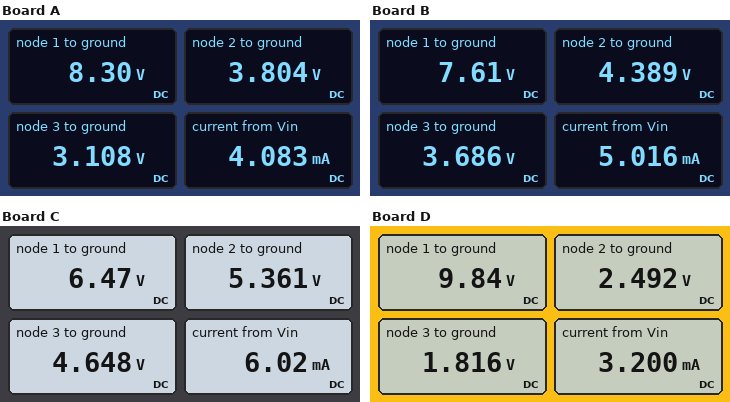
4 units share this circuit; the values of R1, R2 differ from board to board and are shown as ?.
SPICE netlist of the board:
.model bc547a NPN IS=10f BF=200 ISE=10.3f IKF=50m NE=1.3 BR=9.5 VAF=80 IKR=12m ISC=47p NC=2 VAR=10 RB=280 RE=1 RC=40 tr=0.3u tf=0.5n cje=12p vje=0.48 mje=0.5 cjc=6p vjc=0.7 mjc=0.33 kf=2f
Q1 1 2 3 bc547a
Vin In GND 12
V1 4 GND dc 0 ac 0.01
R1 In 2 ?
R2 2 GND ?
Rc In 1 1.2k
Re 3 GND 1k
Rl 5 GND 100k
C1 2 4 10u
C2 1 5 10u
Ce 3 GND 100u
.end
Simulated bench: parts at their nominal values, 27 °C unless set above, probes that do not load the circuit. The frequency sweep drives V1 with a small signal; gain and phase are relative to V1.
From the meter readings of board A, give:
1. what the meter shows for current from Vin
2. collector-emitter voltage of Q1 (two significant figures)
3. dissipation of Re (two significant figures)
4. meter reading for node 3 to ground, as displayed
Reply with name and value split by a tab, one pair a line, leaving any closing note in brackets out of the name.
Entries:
what the meter shows for current from Vin	4.083 mA
collector-emitter voltage of Q1	5.2 V
dissipation of Re	9.7 mW
meter reading for node 3 to ground, as displayed	3.108 V
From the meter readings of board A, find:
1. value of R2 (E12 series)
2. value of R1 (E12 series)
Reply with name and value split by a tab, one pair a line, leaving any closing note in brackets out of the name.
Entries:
value of R2	3.9 kΩ
value of R1	8.2 kΩ
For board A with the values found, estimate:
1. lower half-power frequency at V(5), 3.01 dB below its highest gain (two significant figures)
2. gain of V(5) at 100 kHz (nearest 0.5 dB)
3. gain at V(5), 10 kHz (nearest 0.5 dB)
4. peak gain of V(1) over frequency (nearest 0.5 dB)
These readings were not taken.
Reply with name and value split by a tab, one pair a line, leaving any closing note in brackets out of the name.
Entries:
lower half-power frequency at V(5), 3.01 dB below its highest gain	140 Hz
gain of V(5) at 100 kHz	39.5 dB
gain at V(5), 10 kHz	39.5 dB
peak gain of V(1) over frequency	39.5 dB
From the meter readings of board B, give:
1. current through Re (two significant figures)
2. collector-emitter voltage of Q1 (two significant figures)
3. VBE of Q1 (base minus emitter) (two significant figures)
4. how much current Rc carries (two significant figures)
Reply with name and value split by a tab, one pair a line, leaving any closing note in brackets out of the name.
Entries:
current through Re	3.7 mA
collector-emitter voltage of Q1	3.9 V
VBE of Q1 (base minus emitter)	700 mV
how much current Rc carries	3.7 mA
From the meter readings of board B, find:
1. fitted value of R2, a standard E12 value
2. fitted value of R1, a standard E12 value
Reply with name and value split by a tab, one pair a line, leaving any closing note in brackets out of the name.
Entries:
fitted value of R2, a standard E12 value	3.3 kΩ
fitted value of R1, a standard E12 value	5.6 kΩ
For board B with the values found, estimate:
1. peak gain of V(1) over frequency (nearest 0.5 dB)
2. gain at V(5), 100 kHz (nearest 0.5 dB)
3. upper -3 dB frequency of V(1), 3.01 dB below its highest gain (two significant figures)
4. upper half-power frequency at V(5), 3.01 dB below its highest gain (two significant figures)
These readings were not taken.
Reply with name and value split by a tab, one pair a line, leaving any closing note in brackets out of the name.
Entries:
peak gain of V(1) over frequency	40.5 dB
gain at V(5), 100 kHz	40.5 dB
upper -3 dB frequency of V(1), 3.01 dB below its highest gain	1.3 MHz
upper half-power frequency at V(5), 3.01 dB below its highest gain	1.3 MHz
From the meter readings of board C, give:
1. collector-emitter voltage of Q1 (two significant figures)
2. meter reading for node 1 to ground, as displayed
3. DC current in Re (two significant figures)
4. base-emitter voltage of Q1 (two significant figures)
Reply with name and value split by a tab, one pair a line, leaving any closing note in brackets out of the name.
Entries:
collector-emitter voltage of Q1	1.8 V
meter reading for node 1 to ground, as displayed	6.47 V
DC current in Re	4.6 mA
base-emitter voltage of Q1	710 mV
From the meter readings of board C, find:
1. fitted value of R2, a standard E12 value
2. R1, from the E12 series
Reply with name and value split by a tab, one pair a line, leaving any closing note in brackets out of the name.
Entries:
fitted value of R2, a standard E12 value	3.9 kΩ
R1, from the E12 series	4.7 kΩ
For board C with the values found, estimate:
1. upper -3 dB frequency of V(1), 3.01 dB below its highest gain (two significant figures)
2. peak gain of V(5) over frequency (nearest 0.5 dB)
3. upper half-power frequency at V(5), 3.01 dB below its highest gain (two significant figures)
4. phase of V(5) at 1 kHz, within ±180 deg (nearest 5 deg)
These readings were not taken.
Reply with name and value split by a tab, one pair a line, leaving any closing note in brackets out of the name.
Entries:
upper -3 dB frequency of V(1), 3.01 dB below its highest gain	890 kHz
peak gain of V(5) over frequency	41.5 dB
upper half-power frequency at V(5), 3.01 dB below its highest gain	890 kHz
phase of V(5) at 1 kHz, within ±180 deg	-170 deg
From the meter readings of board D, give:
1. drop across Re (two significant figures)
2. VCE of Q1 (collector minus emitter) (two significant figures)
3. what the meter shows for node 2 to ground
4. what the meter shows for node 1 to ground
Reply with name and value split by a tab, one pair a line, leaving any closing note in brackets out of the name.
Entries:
drop across Re	1.8 V
VCE of Q1 (collector minus emitter)	8.0 V
what the meter shows for node 2 to ground	2.492 V
what the meter shows for node 1 to ground	9.84 V
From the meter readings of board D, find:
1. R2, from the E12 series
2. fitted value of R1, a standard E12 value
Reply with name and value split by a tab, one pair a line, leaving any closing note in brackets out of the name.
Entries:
R2, from the E12 series	1.8 kΩ
fitted value of R1, a standard E12 value	6.8 kΩ
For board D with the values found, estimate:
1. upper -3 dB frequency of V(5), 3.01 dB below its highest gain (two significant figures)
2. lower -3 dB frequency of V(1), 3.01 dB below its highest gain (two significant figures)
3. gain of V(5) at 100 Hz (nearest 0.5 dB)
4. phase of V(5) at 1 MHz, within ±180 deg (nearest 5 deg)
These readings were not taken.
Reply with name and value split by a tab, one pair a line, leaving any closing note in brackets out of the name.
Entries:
upper -3 dB frequency of V(5), 3.01 dB below its highest gain	2.3 MHz
lower -3 dB frequency of V(1), 3.01 dB below its highest gain	97 Hz
gain of V(5) at 100 Hz	33.5 dB
phase of V(5) at 1 MHz, within ±180 deg	155 deg
